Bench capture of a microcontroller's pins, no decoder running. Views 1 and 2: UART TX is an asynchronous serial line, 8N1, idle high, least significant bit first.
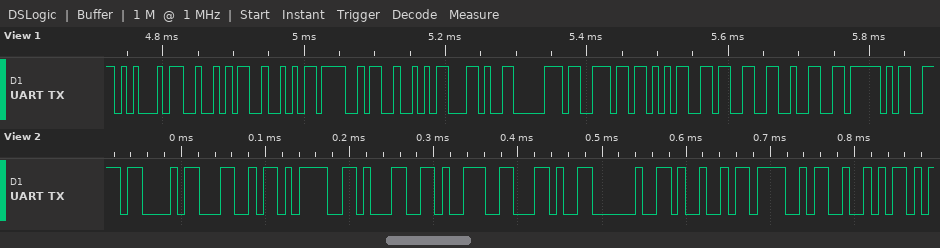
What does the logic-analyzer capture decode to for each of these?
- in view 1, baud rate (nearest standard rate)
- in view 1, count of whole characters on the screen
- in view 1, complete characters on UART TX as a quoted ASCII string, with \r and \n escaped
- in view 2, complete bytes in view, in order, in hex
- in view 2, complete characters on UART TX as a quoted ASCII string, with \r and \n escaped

115200 baud
12
"ERROR,pn532_"
0x43 0x4C 0x3D 0x31 0x39 0x2C 0x20 0x49 0x4F 0x52
"CL=19, IOR"
